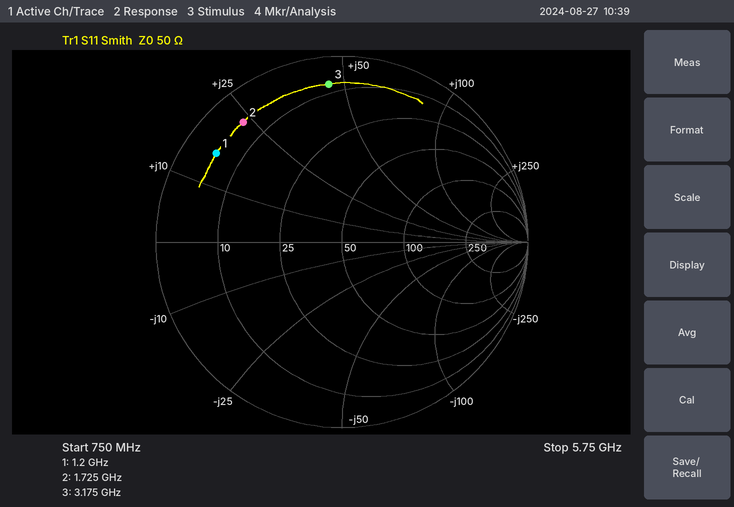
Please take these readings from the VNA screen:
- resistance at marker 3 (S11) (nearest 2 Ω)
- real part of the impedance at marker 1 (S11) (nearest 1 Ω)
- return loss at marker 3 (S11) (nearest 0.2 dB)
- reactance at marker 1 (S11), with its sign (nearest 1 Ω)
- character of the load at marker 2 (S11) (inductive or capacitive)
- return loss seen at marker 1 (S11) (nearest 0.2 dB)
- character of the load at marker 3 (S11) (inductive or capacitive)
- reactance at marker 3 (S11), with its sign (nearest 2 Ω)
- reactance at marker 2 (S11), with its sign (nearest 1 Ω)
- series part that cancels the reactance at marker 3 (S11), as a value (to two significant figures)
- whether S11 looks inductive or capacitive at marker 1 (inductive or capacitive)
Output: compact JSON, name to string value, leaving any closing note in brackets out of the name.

{"resistance at marker 3 (S11)": "8 Ω", "real part of the impedance at marker 1 (S11)": "5 Ω", "return loss at marker 3 (S11)": "1.4 dB", "reactance at marker 1 (S11), with its sign": "+16 Ω", "character of the load at marker 2 (S11)": "inductive", "return loss seen at marker 1 (S11)": "1.6 dB", "character of the load at marker 3 (S11)": "inductive", "reactance at marker 3 (S11), with its sign": "+46 Ω", "reactance at marker 2 (S11), with its sign": "+23 Ω", "series part that cancels the reactance at marker 3 (S11), as a value": "1.1 pF", "whether S11 looks inductive or capacitive at marker 1": "inductive"}
